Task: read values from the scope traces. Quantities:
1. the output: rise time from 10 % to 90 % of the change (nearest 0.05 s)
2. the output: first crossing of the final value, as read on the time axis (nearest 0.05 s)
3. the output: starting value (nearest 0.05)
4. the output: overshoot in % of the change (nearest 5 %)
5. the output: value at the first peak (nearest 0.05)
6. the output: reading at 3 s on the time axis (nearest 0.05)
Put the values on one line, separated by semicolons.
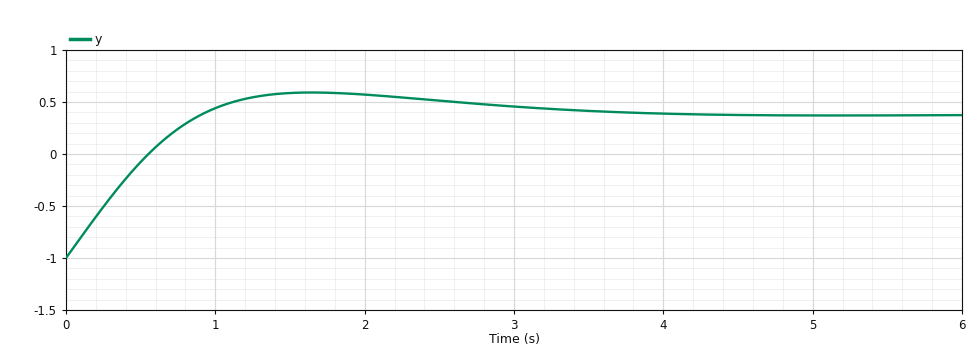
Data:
0.70 s; 0.90 s; -1.00; 15 %; 0.60; 0.45
